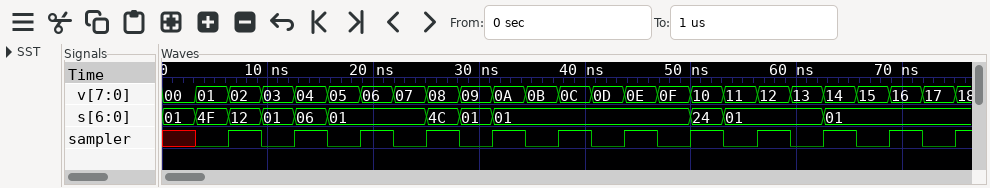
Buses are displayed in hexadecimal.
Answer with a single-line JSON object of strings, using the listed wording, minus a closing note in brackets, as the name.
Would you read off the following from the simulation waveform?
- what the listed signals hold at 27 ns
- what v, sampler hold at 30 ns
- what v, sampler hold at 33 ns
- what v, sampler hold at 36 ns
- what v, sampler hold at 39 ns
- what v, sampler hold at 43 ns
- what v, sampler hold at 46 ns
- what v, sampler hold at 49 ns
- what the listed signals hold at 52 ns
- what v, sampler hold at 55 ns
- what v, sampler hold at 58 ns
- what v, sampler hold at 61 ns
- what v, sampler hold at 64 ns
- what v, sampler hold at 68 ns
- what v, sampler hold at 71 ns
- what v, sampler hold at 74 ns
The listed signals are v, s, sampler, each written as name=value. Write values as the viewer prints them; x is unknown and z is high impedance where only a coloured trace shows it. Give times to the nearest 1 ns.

{"what the listed signals hold at 27 ns": "v=08, s=4C, sampler=1", "what v, sampler hold at 30 ns": "v=09, sampler=0", "what v, sampler hold at 33 ns": "v=0A, sampler=1", "what v, sampler hold at 36 ns": "v=0B, sampler=0", "what v, sampler hold at 39 ns": "v=0C, sampler=1", "what v, sampler hold at 43 ns": "v=0D, sampler=0", "what v, sampler hold at 46 ns": "v=0E, sampler=1", "what v, sampler hold at 49 ns": "v=0F, sampler=0", "what the listed signals hold at 52 ns": "v=10, s=24, sampler=1", "what v, sampler hold at 55 ns": "v=11, sampler=0", "what v, sampler hold at 58 ns": "v=12, sampler=1", "what v, sampler hold at 61 ns": "v=13, sampler=0", "what v, sampler hold at 64 ns": "v=14, sampler=1", "what v, sampler hold at 68 ns": "v=15, sampler=0", "what v, sampler hold at 71 ns": "v=16, sampler=1", "what v, sampler hold at 74 ns": "v=17, sampler=0"}
